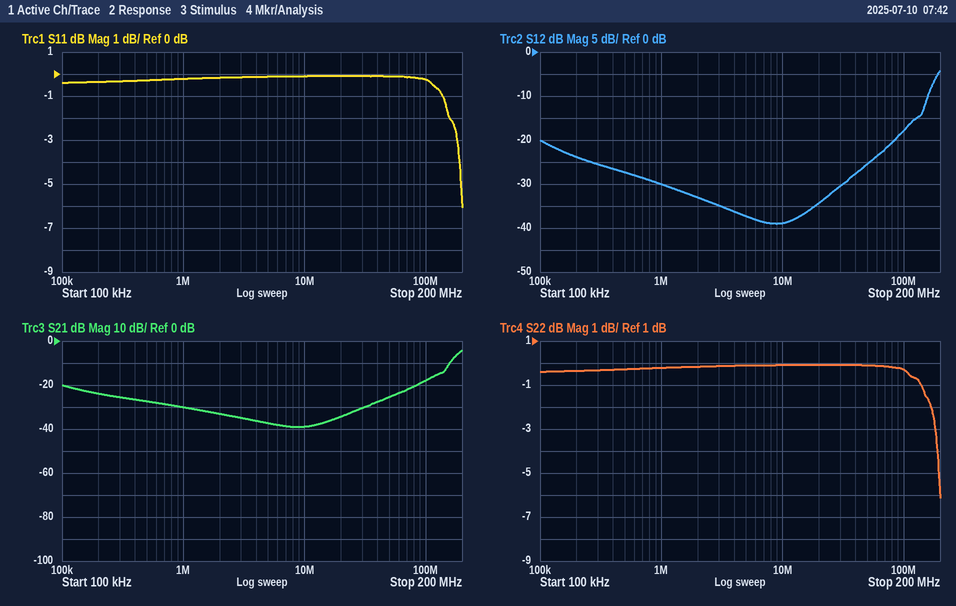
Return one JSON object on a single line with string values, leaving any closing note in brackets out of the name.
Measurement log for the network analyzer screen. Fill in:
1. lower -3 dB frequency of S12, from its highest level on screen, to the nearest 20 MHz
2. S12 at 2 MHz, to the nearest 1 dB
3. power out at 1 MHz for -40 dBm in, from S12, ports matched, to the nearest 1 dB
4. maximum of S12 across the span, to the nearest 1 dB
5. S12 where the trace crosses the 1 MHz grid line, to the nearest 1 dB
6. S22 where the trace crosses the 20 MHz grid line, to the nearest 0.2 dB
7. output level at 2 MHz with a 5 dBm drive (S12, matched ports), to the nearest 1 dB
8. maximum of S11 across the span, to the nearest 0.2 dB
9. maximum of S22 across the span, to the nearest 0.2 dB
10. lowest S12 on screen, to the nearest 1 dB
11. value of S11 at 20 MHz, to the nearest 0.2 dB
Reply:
{"lower -3 dB frequency of S12, from its highest level on screen, to the nearest 20 MHz": "180 MHz", "S12 at 2 MHz, to the nearest 1 dB": "-33 dB", "power out at 1 MHz for -40 dBm in, from S12, ports matched, to the nearest 1 dB": "-70 dBm", "maximum of S12 across the span, to the nearest 1 dB": "-4 dB", "S12 where the trace crosses the 1 MHz grid line, to the nearest 1 dB": "-30 dB", "S22 where the trace crosses the 20 MHz grid line, to the nearest 0.2 dB": "0.0 dB", "output level at 2 MHz with a 5 dBm drive (S12, matched ports), to the nearest 1 dB": "-28 dBm", "maximum of S11 across the span, to the nearest 0.2 dB": "0.0 dB", "maximum of S22 across the span, to the nearest 0.2 dB": "0.0 dB", "lowest S12 on screen, to the nearest 1 dB": "-39 dB", "value of S11 at 20 MHz, to the nearest 0.2 dB": "0.0 dB"}
